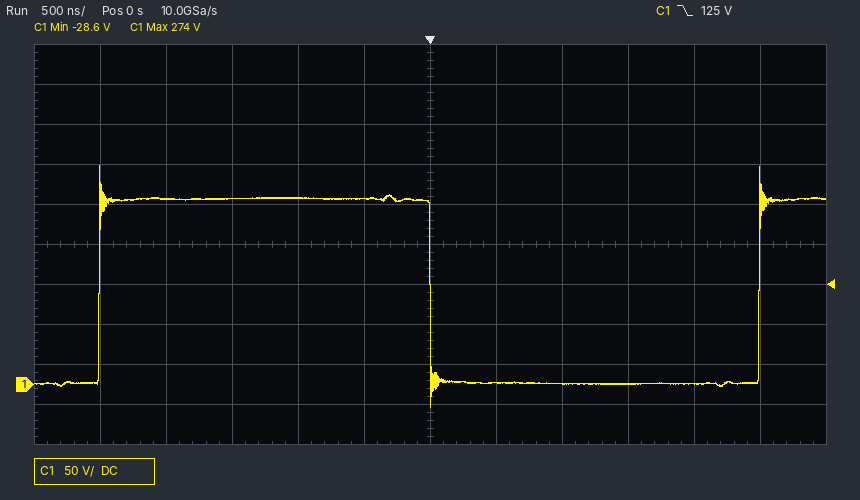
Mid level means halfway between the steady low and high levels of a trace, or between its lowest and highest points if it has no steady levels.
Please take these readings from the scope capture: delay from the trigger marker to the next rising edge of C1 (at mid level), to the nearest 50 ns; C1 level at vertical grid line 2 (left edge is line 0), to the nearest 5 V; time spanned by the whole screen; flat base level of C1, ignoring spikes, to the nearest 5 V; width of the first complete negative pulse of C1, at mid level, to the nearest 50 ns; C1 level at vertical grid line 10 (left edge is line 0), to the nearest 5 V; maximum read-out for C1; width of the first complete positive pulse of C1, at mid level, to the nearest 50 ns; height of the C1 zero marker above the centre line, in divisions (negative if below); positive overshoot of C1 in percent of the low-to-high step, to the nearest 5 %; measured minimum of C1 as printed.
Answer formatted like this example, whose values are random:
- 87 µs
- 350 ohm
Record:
- 2.50 µs
- 230 V
- 6 µs
- 0 V
- 2.50 µs
- 0 V
- 274 V
- 2.50 µs
- -3.5 div
- 20 %
- -28.6 V
